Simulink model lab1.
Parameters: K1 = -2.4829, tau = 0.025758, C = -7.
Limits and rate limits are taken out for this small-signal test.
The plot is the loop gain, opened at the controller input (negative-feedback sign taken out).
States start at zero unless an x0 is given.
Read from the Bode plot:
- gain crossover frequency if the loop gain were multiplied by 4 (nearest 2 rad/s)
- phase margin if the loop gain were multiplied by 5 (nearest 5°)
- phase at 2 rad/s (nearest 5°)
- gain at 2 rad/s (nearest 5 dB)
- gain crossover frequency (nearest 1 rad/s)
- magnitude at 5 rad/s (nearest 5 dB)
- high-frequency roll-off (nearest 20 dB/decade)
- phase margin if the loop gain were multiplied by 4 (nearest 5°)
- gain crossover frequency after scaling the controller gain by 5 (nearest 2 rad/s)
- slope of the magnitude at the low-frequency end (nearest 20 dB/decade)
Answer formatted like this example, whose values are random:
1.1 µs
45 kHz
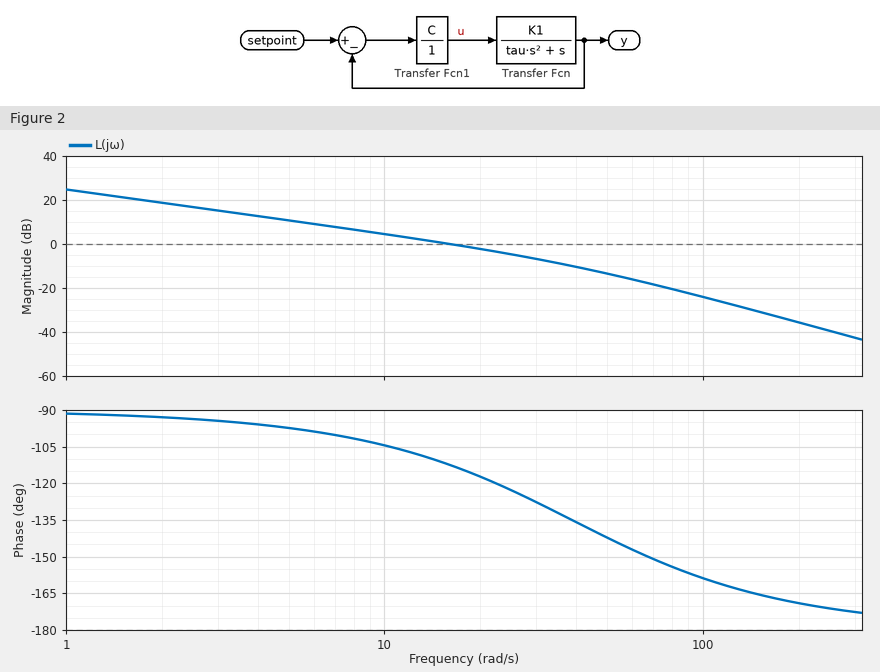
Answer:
46 rad/s
35°
-95°
20 dB
16 rad/s
10 dB
-40 dB/decade
40°
52 rad/s
-20 dB/decade
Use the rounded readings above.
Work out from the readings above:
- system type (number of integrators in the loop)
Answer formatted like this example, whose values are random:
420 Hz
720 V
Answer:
1
